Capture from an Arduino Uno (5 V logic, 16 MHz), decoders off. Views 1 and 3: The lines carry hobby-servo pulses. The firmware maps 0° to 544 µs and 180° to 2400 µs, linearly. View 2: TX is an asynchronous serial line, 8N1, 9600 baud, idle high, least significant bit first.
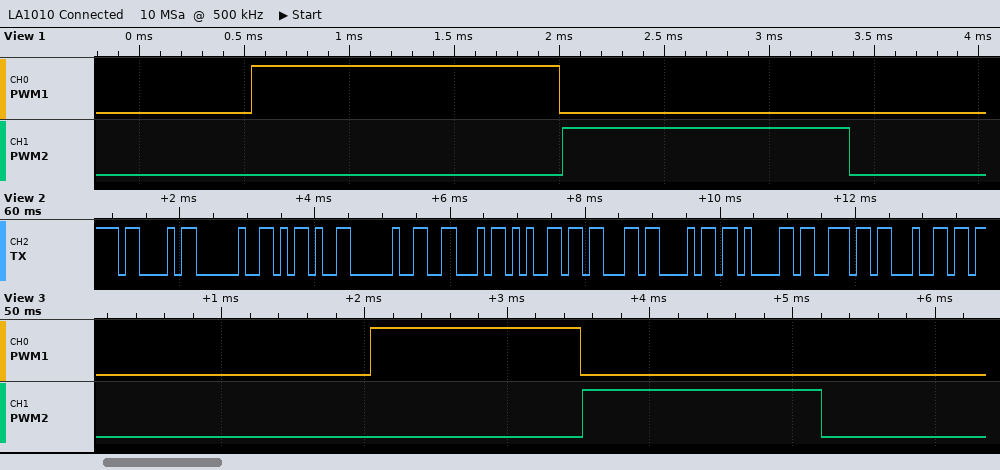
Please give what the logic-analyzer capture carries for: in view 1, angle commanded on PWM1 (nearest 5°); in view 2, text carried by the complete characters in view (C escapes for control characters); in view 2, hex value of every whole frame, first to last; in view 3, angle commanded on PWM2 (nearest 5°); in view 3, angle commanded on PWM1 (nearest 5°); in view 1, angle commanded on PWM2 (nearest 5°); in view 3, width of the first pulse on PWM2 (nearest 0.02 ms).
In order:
90°
"C - Fechand"
43 20 2D 20 46 65 63 68 61 6E 64
110°
90°
80°
1.68 ms
